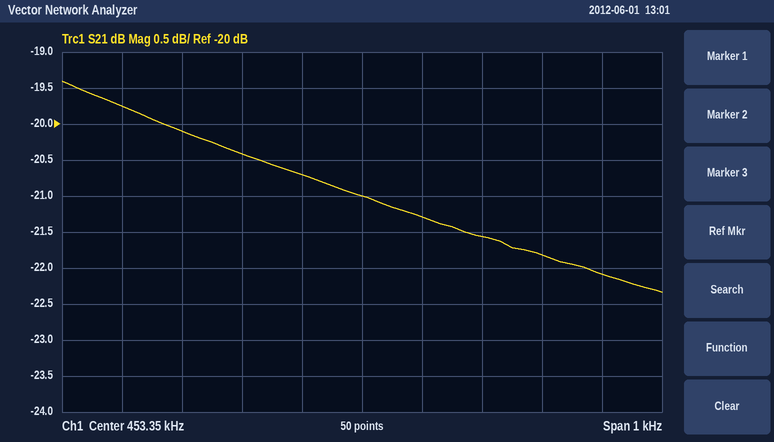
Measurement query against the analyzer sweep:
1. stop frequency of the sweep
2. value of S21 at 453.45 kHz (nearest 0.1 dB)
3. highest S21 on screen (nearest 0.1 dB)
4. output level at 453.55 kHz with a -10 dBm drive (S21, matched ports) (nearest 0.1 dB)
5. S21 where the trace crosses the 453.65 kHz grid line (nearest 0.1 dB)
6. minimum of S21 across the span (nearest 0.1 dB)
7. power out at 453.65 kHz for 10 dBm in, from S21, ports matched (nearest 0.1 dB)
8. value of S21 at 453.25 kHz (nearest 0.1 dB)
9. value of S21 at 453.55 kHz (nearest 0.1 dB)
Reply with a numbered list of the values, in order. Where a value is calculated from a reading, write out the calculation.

1. 453.85 kHz
2. -21.3 dB
3. -19.4 dB
4. -10 dBm + (-21.6 dB) = -31.6 dBm
5. -21.8 dB
6. -22.3 dB
7. 10 dBm + (-21.8 dB) = -11.8 dBm
8. -20.7 dB
9. -21.6 dB
